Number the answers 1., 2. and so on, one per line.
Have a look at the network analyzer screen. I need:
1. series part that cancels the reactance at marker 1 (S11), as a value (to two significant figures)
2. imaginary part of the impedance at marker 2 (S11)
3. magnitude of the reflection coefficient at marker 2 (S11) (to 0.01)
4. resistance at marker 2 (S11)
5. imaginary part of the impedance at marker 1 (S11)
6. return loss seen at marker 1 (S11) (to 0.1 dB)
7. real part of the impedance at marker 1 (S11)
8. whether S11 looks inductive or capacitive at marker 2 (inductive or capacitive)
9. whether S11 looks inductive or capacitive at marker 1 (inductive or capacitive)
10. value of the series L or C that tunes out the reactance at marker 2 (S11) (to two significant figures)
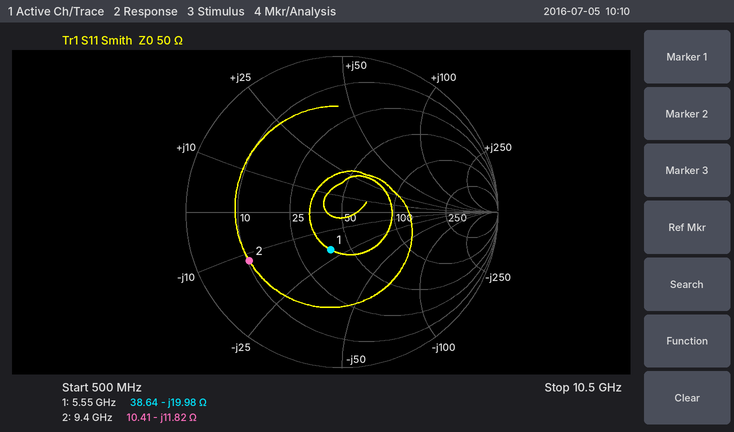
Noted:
1. 570 pH
2. -11.82 Ω
3. 0.67
4. 10.41 Ω
5. -19.98 Ω
6. 11.9 dB
7. 38.64 Ω
8. capacitive
9. capacitive
10. 200 pH
